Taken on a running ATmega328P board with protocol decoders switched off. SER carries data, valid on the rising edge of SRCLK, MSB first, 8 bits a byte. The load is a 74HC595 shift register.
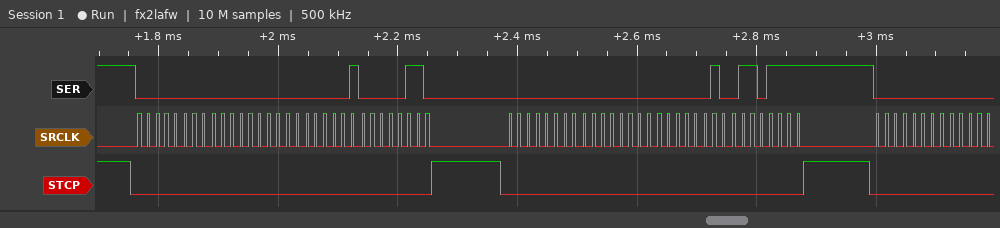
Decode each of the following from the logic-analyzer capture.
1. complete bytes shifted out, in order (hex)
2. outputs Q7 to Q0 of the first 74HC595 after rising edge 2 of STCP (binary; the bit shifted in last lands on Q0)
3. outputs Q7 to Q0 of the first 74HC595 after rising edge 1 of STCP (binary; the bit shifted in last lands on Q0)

00 00 01 06 00 00 02 6F 00
01101111
00000110
